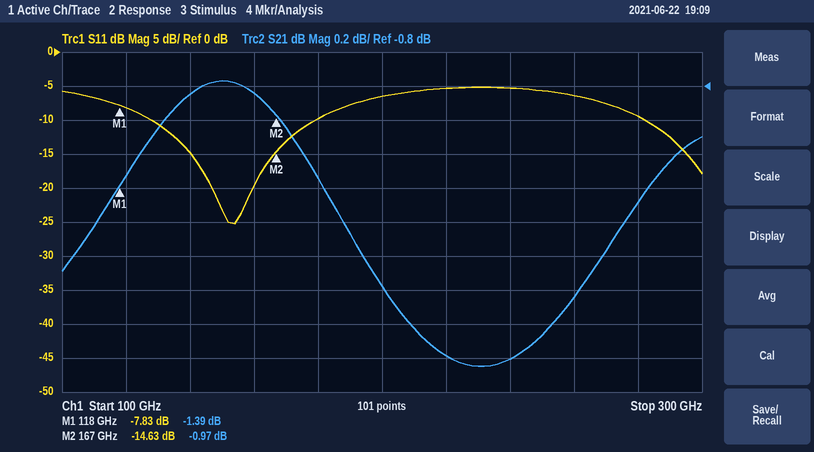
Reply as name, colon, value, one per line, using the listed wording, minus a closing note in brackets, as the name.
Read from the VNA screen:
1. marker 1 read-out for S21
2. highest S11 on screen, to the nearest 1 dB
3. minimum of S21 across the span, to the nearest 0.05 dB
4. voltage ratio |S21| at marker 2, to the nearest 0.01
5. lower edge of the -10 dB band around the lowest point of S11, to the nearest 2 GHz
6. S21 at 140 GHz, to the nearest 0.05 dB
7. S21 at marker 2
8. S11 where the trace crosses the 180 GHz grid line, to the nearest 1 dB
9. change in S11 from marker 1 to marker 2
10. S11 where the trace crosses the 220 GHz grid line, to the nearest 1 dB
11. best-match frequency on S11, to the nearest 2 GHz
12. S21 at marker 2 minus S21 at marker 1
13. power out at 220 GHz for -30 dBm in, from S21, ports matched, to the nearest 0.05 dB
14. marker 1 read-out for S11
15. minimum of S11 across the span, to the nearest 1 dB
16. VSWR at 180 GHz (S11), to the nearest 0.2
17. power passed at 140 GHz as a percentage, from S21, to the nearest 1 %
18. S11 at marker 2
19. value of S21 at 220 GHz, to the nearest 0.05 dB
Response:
marker 1 read-out for S21: -1.39 dB
highest S11 on screen, to the nearest 1 dB: -5 dB
minimum of S21 across the span, to the nearest 0.05 dB: -2.45 dB
voltage ratio |S21| at marker 2, to the nearest 0.01: 0.89
lower edge of the -10 dB band around the lowest point of S11, to the nearest 2 GHz: 128 GHz
S21 at 140 GHz, to the nearest 0.05 dB: -0.85 dB
S21 at marker 2: -0.97 dB
S11 where the trace crosses the 180 GHz grid line, to the nearest 1 dB: -10 dB
change in S11 from marker 1 to marker 2: -6.80 dB
S11 where the trace crosses the 220 GHz grid line, to the nearest 1 dB: -5 dB
best-match frequency on S11, to the nearest 2 GHz: 154 GHz
S21 at marker 2 minus S21 at marker 1: 0.42 dB
power out at 220 GHz for -30 dBm in, from S21, ports matched, to the nearest 0.05 dB: -32.40 dBm
marker 1 read-out for S11: -7.83 dB
minimum of S11 across the span, to the nearest 1 dB: -25 dB
VSWR at 180 GHz (S11), to the nearest 0.2: 2.0
power passed at 140 GHz as a percentage, from S21, to the nearest 1 %: 82 %
S11 at marker 2: -14.63 dB
value of S21 at 220 GHz, to the nearest 0.05 dB: -2.40 dB
